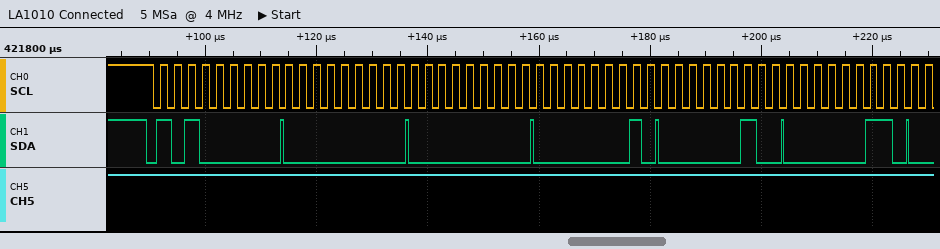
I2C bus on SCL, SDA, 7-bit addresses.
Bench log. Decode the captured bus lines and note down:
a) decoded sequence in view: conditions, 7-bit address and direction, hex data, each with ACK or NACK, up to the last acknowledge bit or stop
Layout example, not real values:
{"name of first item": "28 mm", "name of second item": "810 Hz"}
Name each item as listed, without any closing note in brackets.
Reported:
{"decoded sequence in view: conditions, 7-bit address and direction, hex data, each with ACK or NACK, up to the last acknowledge bit or stop": "start, address 50 write ACK, 00 ACK, 00 ACK, 01 ACK, 02 ACK, 03 ACK"}
